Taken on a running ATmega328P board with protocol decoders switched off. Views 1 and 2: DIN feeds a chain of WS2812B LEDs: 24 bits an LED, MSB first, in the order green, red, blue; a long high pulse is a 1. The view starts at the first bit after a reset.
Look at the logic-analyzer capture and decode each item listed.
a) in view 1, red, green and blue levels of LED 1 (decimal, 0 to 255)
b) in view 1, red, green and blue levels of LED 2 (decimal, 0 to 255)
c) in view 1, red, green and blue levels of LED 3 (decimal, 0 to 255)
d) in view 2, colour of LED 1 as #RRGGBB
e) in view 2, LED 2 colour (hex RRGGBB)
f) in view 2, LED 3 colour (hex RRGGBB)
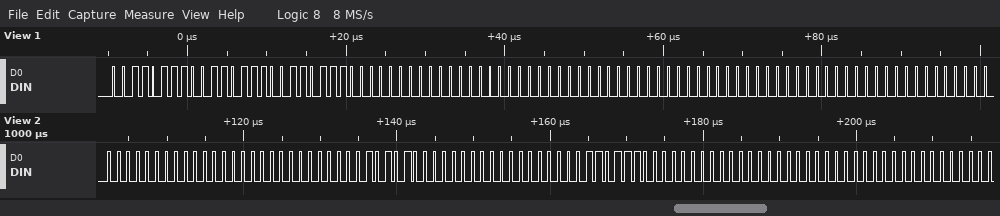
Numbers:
55, 55, 55
0, 0, 0
0, 0, 0
#000000
#001500
#003700
